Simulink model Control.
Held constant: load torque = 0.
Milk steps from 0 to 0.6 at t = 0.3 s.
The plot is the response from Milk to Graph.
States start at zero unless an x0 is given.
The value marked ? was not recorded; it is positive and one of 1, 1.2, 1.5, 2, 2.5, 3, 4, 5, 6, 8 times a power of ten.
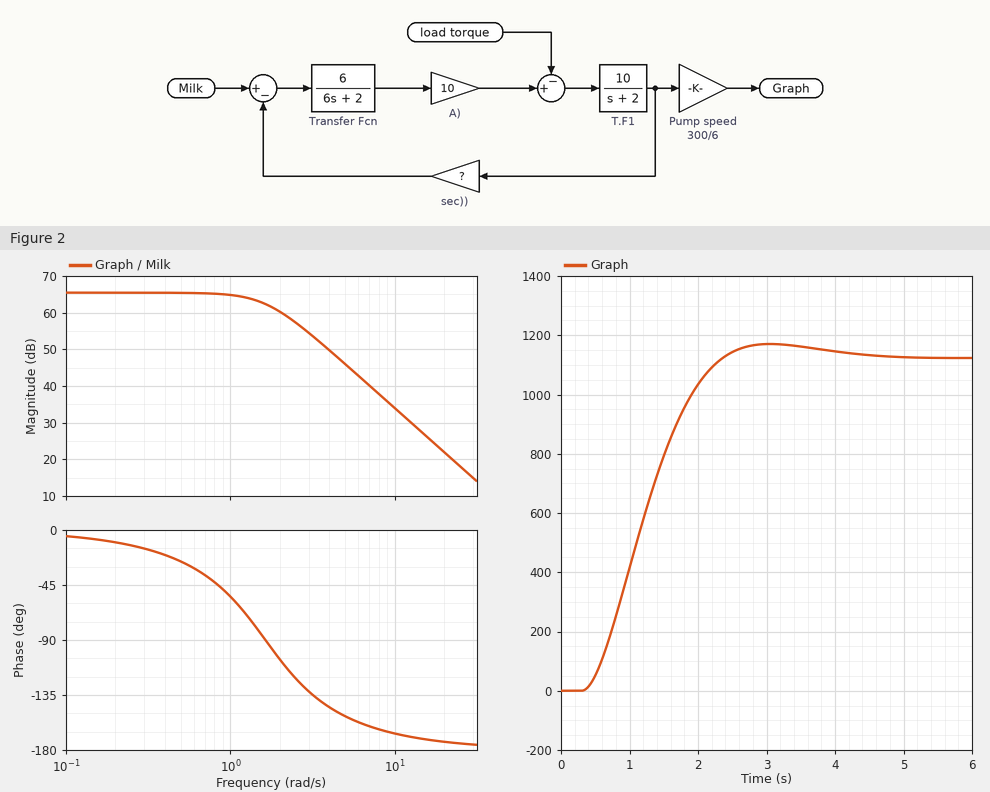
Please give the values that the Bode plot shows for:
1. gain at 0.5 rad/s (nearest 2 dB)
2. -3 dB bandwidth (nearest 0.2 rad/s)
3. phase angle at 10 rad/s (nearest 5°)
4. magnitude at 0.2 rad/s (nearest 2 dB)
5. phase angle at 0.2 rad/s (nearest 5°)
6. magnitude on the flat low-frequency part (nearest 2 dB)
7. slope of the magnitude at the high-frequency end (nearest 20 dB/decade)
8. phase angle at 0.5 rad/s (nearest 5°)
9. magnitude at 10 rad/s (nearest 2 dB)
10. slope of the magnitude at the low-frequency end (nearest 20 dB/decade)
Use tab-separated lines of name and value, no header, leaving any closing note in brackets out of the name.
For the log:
gain at 0.5 rad/s	66 dB
-3 dB bandwidth	1.6 rad/s
phase angle at 10 rad/s	-165°
magnitude at 0.2 rad/s	66 dB
phase angle at 0.2 rad/s	-10°
magnitude on the flat low-frequency part	66 dB
slope of the magnitude at the high-frequency end	-40 dB/decade
phase angle at 0.5 rad/s	-25°
magnitude at 10 rad/s	34 dB
slope of the magnitude at the low-frequency end	0 dB/decade
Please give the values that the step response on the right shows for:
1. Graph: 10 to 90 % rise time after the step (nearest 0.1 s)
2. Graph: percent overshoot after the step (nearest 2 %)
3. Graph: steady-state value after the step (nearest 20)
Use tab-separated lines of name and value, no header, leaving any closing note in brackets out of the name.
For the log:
Graph: 10 to 90 % rise time after the step	1.3 s
Graph: percent overshoot after the step	4 %
Graph: steady-state value after the step	1120
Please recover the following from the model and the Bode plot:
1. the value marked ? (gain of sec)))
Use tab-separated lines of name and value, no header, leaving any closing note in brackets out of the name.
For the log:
the value marked ? (gain of sec)))	0.02
